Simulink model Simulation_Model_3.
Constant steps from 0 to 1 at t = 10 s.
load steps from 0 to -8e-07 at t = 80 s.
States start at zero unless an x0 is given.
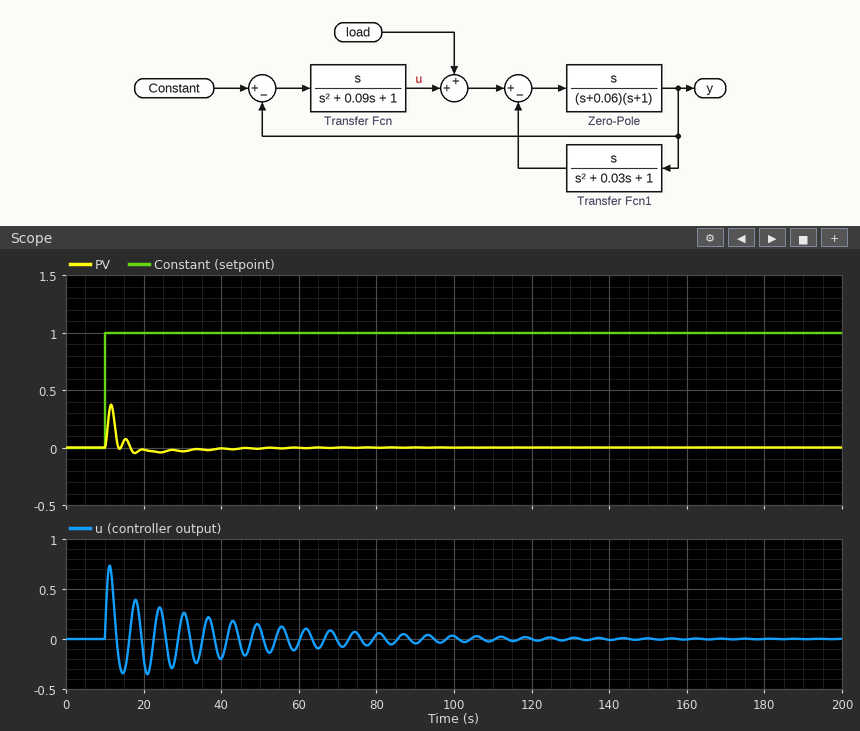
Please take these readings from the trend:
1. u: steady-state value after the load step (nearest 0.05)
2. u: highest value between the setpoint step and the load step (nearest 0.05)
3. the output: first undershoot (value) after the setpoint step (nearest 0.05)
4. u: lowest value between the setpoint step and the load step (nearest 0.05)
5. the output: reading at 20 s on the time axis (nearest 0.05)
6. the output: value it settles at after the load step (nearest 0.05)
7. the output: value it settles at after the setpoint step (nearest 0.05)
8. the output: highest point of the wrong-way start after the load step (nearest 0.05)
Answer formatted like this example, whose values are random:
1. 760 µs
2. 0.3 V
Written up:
1. 0.00
2. 0.75
3. 0.00
4. -0.35
5. 0.00
6. 0.00
7. 0.00
8. 0.00
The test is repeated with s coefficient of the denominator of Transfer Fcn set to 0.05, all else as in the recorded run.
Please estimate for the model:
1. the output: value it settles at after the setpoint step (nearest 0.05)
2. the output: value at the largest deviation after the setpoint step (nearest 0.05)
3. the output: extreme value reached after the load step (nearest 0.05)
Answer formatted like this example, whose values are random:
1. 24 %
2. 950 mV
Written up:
1. 0.00
2. 0.40
3. 0.00
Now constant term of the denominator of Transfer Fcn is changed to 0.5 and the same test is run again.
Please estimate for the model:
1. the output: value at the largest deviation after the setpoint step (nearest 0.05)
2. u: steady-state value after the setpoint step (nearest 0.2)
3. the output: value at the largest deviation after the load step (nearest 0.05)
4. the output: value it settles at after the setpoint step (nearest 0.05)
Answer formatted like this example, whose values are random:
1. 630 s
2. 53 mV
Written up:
1. 0.45
2. 0.0
3. 0.00
4. 0.00
